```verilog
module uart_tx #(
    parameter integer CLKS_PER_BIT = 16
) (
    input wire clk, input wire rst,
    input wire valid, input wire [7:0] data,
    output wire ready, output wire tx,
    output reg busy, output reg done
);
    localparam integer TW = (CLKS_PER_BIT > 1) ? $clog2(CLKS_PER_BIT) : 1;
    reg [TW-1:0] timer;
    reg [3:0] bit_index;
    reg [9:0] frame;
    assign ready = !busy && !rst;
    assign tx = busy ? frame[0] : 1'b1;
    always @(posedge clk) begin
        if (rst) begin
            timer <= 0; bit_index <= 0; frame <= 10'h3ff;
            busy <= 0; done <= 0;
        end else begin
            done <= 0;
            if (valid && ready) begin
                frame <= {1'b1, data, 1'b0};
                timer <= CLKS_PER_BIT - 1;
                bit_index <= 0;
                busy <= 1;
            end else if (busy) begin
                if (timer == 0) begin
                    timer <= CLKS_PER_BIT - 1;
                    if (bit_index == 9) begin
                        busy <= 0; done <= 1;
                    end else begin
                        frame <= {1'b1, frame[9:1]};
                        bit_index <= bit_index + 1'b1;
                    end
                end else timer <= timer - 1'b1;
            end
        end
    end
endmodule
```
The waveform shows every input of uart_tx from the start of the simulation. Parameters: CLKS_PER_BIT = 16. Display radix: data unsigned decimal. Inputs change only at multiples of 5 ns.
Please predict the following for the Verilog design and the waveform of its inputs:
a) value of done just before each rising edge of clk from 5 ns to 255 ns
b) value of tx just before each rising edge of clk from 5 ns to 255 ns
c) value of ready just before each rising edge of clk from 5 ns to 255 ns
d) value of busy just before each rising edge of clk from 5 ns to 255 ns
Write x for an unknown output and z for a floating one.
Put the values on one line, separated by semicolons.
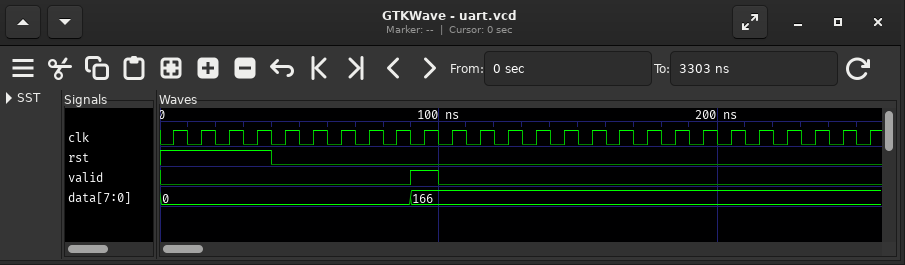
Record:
x 0 0 0 0 0 0 0 0 0 0 0 0 0 0 0 0 0 0 0 0 0 0 0 0 0; x 1 1 1 1 1 1 1 1 1 0 0 0 0 0 0 0 0 0 0 0 0 0 0 0 0; 0 0 0 0 1 1 1 1 1 1 0 0 0 0 0 0 0 0 0 0 0 0 0 0 0 0; x 0 0 0 0 0 0 0 0 0 1 1 1 1 1 1 1 1 1 1 1 1 1 1 1 1
